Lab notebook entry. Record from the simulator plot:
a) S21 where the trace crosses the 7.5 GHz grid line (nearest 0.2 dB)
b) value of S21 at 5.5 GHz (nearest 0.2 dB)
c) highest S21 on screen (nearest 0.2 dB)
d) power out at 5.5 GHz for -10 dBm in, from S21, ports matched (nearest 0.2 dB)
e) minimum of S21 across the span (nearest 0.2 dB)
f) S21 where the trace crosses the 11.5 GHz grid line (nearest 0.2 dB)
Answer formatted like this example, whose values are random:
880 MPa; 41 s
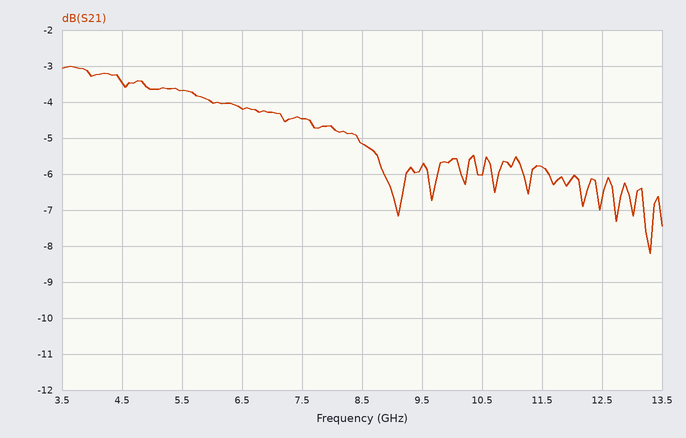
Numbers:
-4.4 dB; -3.6 dB; -3.0 dB; -13.6 dBm; -8.2 dB; -5.8 dB
